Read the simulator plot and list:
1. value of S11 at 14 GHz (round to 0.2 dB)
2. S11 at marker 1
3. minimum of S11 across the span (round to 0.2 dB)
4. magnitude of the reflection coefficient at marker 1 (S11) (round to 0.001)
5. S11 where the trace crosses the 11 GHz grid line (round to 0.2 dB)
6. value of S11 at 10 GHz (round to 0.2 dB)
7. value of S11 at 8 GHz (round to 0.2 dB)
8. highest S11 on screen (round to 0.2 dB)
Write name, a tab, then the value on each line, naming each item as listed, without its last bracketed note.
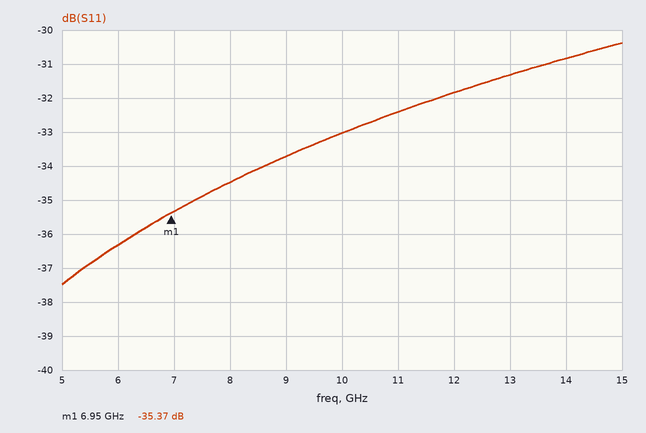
value of S11 at 14 GHz	-30.8 dB
S11 at marker 1	-35.37 dB
minimum of S11 across the span	-37.4 dB
magnitude of the reflection coefficient at marker 1 (S11)	0.017
S11 where the trace crosses the 11 GHz grid line	-32.4 dB
value of S11 at 10 GHz	-33.0 dB
value of S11 at 8 GHz	-34.4 dB
highest S11 on screen	-30.4 dB
